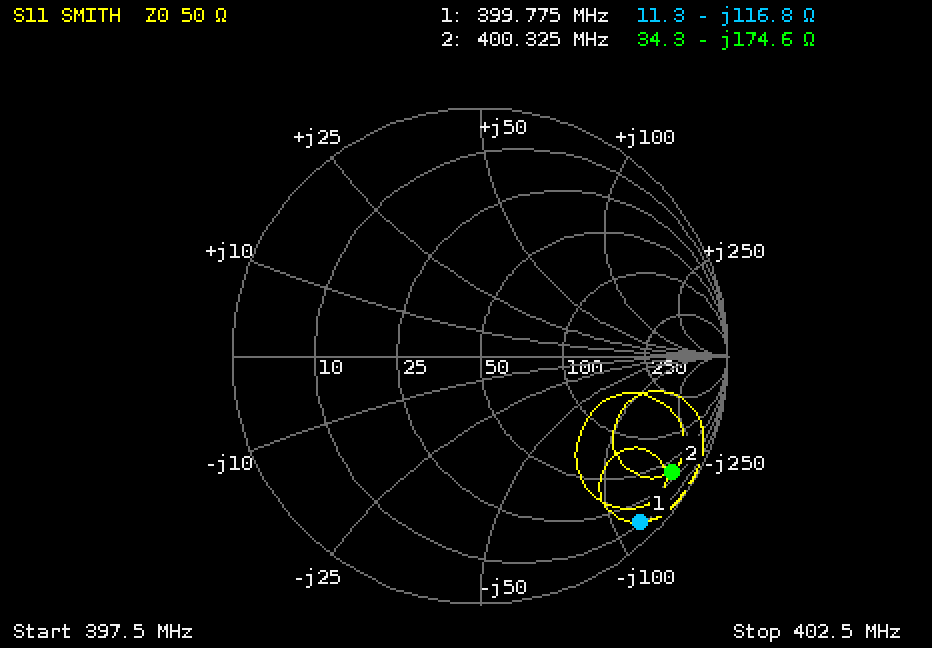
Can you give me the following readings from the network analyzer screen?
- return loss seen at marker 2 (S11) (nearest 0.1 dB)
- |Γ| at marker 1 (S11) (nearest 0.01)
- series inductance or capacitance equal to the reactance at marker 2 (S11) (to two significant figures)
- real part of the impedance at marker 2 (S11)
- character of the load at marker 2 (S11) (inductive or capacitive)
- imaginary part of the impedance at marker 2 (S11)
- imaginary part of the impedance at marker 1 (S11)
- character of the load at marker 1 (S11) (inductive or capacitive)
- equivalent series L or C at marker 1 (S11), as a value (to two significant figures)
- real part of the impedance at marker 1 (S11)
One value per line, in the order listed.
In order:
0.9 dB
0.93
2.3 pF
34.3 Ω
capacitive
-174.6 Ω
-116.8 Ω
capacitive
3.4 pF
11.3 Ω
